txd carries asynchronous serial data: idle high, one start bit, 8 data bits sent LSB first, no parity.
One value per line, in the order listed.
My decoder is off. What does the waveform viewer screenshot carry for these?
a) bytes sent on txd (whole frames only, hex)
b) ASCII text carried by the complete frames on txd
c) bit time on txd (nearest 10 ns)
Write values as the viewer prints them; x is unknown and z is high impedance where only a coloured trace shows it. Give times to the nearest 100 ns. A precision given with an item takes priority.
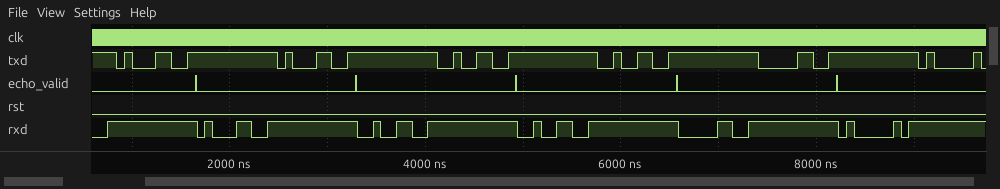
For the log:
31, 31, 32, 32, 30
"11220"
80 ns
